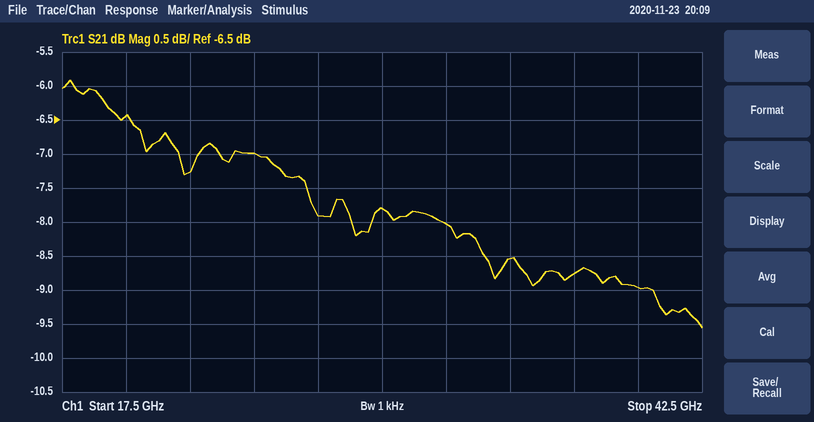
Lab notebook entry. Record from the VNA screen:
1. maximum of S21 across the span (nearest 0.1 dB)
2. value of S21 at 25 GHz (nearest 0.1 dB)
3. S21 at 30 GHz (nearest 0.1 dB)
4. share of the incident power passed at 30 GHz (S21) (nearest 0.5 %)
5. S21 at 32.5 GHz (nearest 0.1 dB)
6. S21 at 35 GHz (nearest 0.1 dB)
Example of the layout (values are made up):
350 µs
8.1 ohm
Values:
-5.9 dB
-7.0 dB
-7.8 dB
16.5 %
-8.0 dB
-8.5 dB
